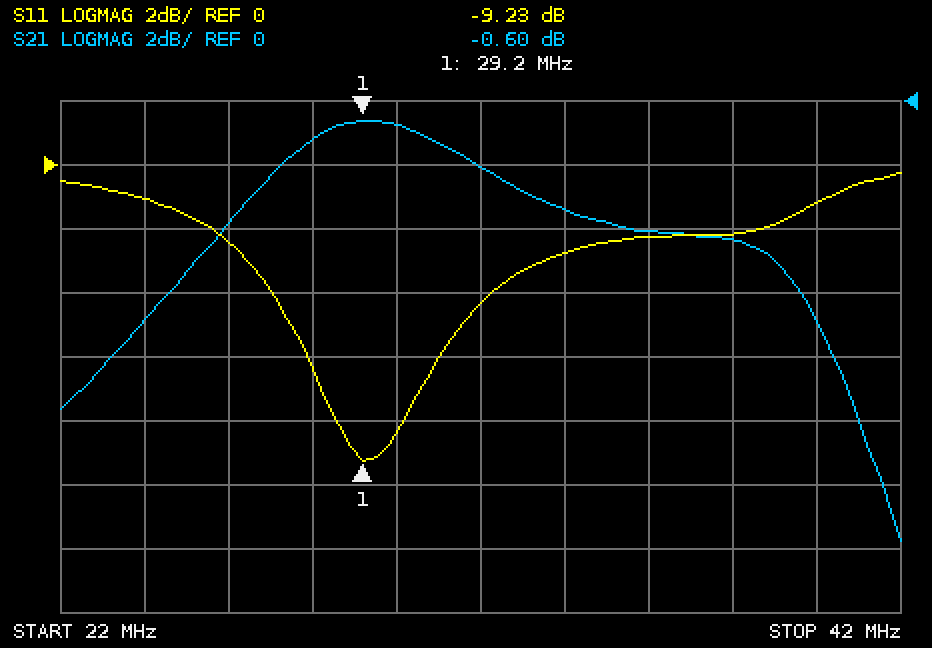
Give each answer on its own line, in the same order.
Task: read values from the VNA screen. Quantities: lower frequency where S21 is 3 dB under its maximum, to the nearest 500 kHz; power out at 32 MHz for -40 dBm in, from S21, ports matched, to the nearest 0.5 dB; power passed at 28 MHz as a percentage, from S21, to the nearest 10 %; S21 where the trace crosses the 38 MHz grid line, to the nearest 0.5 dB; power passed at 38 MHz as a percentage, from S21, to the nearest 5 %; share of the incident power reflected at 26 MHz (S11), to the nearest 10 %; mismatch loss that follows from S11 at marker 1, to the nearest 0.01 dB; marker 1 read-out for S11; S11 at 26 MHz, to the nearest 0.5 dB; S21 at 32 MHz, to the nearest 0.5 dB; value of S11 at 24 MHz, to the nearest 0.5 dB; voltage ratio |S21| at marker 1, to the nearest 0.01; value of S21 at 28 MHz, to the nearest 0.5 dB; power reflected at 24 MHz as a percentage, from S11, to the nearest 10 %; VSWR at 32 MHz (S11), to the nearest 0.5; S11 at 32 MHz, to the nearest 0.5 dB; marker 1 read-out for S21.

26.0 MHz
-42.0 dBm
80 %
-4.5 dB
35 %
60 %
0.55 dB
-9.23 dB
-2.5 dB
-2.0 dB
-1.0 dB
0.93
-1.0 dB
80 %
4.0
-4.5 dB
-0.60 dB
